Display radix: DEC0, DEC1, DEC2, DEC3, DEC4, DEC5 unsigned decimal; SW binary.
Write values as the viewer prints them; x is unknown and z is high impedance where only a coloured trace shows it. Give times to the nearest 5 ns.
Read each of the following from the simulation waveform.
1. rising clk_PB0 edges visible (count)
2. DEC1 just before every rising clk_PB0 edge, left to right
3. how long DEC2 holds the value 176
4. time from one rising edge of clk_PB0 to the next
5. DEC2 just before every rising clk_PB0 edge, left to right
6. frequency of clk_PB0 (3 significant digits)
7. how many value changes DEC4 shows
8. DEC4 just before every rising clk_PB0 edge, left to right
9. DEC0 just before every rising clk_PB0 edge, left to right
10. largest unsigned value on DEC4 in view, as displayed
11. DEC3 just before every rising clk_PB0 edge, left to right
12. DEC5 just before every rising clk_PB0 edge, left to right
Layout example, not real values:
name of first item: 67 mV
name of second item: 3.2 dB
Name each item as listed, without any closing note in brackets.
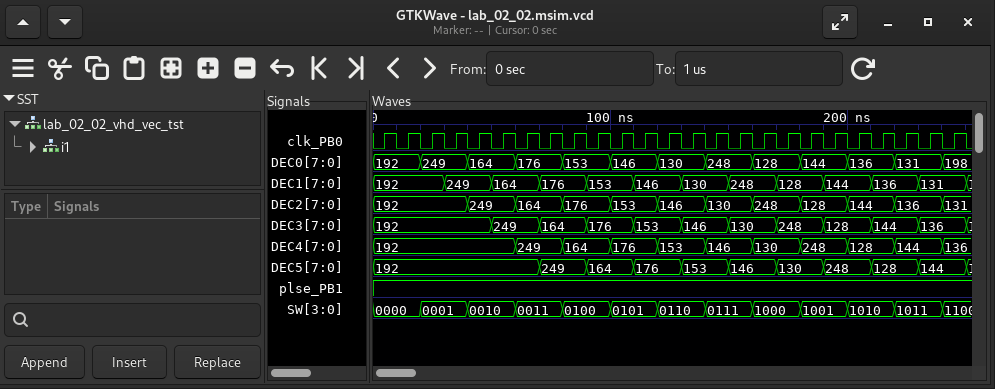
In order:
rising clk_PB0 edges visible: 25
DEC1 just before every rising clk_PB0 edge, left to right: 192, 192, 192, 249, 249, 164, 164, 176, 176, 153, 153, 146, 146, 130, 130, 248, 248, 128, 128, 144, 144, 136, 136, 131, 131
how long DEC2 holds the value 176: 20 ns
time from one rising edge of clk_PB0 to the next: 10 ns
DEC2 just before every rising clk_PB0 edge, left to right: 192, 192, 192, 192, 249, 249, 164, 164, 176, 176, 153, 153, 146, 146, 130, 130, 248, 248, 128, 128, 144, 144, 136, 136, 131
frequency of clk_PB0: 100 MHz
how many value changes DEC4 shows: 10
DEC4 just before every rising clk_PB0 edge, left to right: 192, 192, 192, 192, 192, 192, 249, 249, 164, 164, 176, 176, 153, 153, 146, 146, 130, 130, 248, 248, 128, 128, 144, 144, 136
DEC0 just before every rising clk_PB0 edge, left to right: 192, 192, 249, 249, 164, 164, 176, 176, 153, 153, 146, 146, 130, 130, 248, 248, 128, 128, 144, 144, 136, 136, 131, 131, 198
largest unsigned value on DEC4 in view, as displayed: 249
DEC3 just before every rising clk_PB0 edge, left to right: 192, 192, 192, 192, 192, 249, 249, 164, 164, 176, 176, 153, 153, 146, 146, 130, 130, 248, 248, 128, 128, 144, 144, 136, 136
DEC5 just before every rising clk_PB0 edge, left to right: 192, 192, 192, 192, 192, 192, 192, 249, 249, 164, 164, 176, 176, 153, 153, 146, 146, 130, 130, 248, 248, 128, 128, 144, 144
